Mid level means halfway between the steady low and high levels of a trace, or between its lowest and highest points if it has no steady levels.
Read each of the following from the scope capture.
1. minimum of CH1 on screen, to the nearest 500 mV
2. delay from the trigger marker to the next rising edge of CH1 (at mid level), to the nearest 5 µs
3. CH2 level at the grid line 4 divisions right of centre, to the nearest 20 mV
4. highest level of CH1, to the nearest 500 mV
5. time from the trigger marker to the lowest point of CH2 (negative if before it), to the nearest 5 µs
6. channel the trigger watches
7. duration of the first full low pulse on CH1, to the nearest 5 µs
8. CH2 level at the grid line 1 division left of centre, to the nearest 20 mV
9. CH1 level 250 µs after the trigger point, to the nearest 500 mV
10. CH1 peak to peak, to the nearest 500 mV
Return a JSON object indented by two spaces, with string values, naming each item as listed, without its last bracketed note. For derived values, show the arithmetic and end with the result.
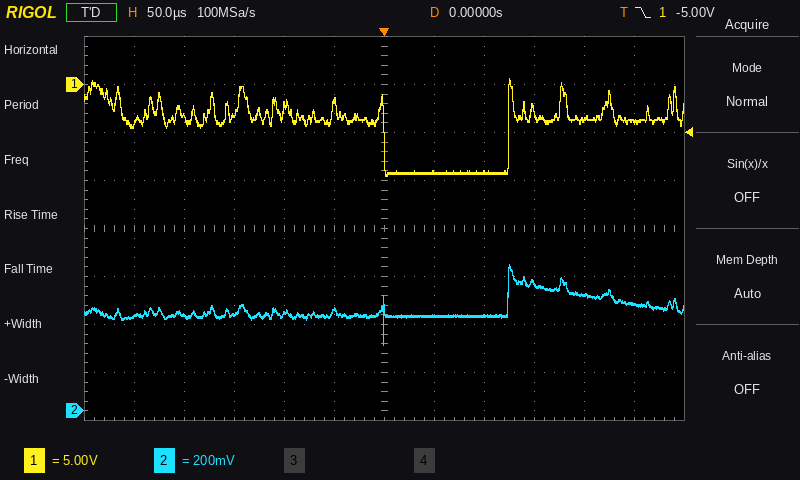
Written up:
{
  "minimum of CH1 on screen, to the nearest 500 mV": "-9.5 V",
  "delay from the trigger marker to the next rising edge of CH1 (at mid level), to the nearest 5 µs": "125 µs",
  "CH2 level at the grid line 4 divisions right of centre, to the nearest 20 mV": "480 mV",
  "highest level of CH1, to the nearest 500 mV": "500 mV",
  "time from the trigger marker to the lowest point of CH2 (negative if before it), to the nearest 5 µs": "0 µs",
  "channel the trigger watches": "CH1",
  "duration of the first full low pulse on CH1, to the nearest 5 µs": "125 µs",
  "CH2 level at the grid line 1 division left of centre, to the nearest 20 mV": "420 mV",
  "CH1 level 250 µs after the trigger point, to the nearest 500 mV": "-4.0 V",
  "CH1 peak to peak, to the nearest 500 mV": "500 mV − (-9.5 V) = 10.0 V"
}
